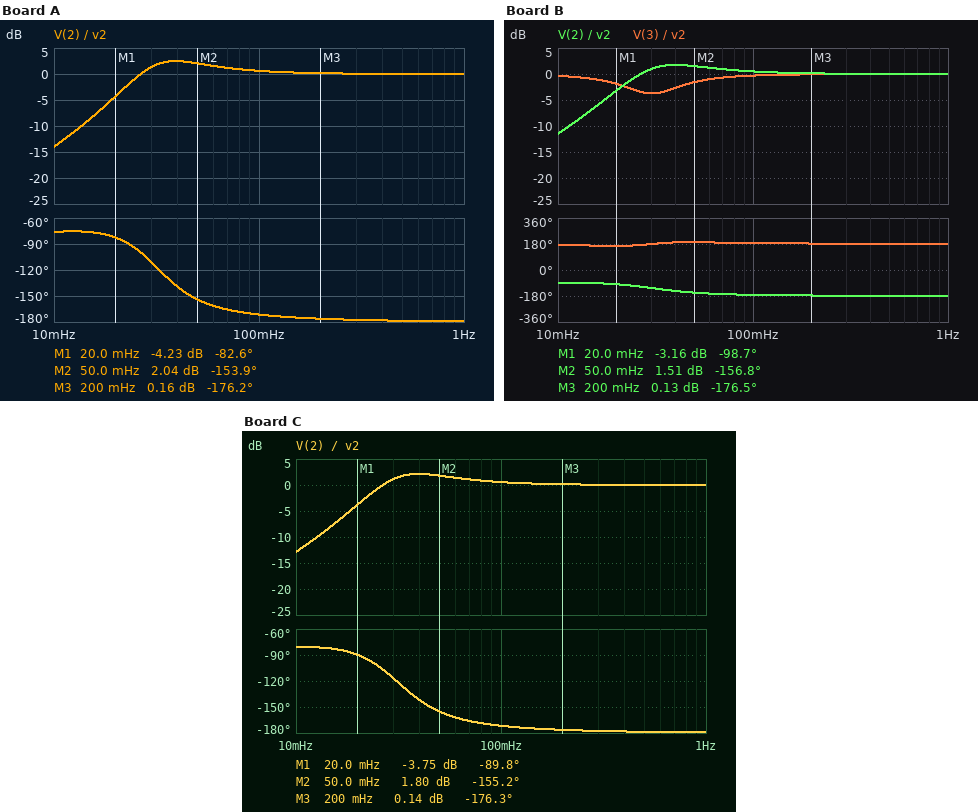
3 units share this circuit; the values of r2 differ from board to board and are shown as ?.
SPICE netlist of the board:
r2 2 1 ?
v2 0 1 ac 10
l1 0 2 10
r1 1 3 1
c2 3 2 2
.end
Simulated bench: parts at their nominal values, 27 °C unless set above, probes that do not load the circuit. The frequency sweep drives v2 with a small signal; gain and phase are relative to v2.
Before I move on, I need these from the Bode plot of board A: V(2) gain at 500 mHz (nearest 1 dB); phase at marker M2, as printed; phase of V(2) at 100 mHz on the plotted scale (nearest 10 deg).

0 dB
-153.9 deg
-170 deg
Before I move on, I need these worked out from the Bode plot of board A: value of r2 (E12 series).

3.9 Ω
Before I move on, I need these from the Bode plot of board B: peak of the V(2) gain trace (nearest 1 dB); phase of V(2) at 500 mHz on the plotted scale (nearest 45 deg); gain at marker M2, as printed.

2 dB
-180 deg
1.51 dB
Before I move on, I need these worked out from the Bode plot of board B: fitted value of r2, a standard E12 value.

2.7 Ω
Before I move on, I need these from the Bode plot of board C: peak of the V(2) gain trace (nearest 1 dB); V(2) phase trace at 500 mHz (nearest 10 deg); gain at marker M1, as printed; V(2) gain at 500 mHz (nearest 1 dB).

2 dB
-180 deg
-3.75 dB
0 dB
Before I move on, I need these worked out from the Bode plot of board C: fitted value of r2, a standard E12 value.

3.3 Ω
